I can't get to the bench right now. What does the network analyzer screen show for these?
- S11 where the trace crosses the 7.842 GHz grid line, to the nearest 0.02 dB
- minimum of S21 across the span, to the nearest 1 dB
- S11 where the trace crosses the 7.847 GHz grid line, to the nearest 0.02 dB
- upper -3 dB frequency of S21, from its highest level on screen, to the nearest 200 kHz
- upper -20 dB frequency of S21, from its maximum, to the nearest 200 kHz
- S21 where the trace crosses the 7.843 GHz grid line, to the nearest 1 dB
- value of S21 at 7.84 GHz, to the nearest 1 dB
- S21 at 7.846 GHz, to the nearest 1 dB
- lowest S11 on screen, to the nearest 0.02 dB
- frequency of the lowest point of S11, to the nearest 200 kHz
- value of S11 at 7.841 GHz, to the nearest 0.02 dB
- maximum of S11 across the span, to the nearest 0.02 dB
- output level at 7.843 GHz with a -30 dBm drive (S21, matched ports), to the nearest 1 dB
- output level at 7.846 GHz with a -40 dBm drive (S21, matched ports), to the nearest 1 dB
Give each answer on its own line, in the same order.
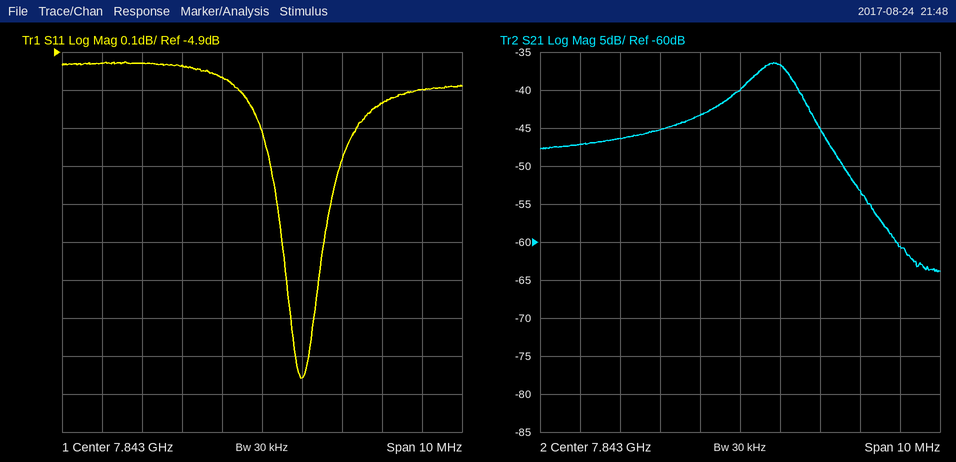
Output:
-4.96 dB
-64 dB
-5.00 dB
7.8444 GHz
7.8464 GHz
-40 dB
-46 dB
-53 dB
-5.76 dB
7.8440 GHz
-4.94 dB
-4.92 dB
-70 dBm
-93 dBm
